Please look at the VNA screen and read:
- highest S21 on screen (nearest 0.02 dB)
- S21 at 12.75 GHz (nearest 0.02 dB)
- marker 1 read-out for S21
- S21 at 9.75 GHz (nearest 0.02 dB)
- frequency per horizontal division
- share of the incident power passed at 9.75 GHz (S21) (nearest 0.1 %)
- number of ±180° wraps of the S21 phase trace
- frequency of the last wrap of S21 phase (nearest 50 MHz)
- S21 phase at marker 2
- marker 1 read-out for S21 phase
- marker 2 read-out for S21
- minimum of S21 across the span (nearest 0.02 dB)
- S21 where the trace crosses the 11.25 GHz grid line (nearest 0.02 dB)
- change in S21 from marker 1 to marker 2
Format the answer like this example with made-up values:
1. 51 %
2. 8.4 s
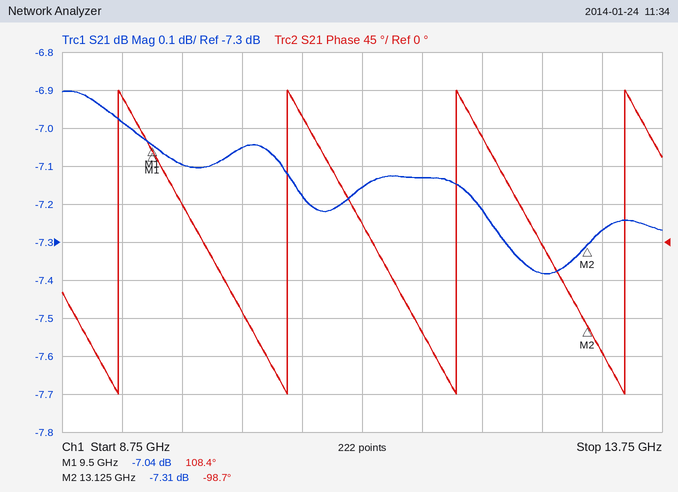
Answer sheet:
1. -6.90 dB
2. -7.38 dB
3. -7.04 dB
4. -7.10 dB
5. 500 MHz
6. 19.5 %
7. 4
8. 13.45 GHz
9. -98.7°
10. 108.4°
11. -7.31 dB
12. -7.38 dB
13. -7.16 dB
14. -0.27 dB
